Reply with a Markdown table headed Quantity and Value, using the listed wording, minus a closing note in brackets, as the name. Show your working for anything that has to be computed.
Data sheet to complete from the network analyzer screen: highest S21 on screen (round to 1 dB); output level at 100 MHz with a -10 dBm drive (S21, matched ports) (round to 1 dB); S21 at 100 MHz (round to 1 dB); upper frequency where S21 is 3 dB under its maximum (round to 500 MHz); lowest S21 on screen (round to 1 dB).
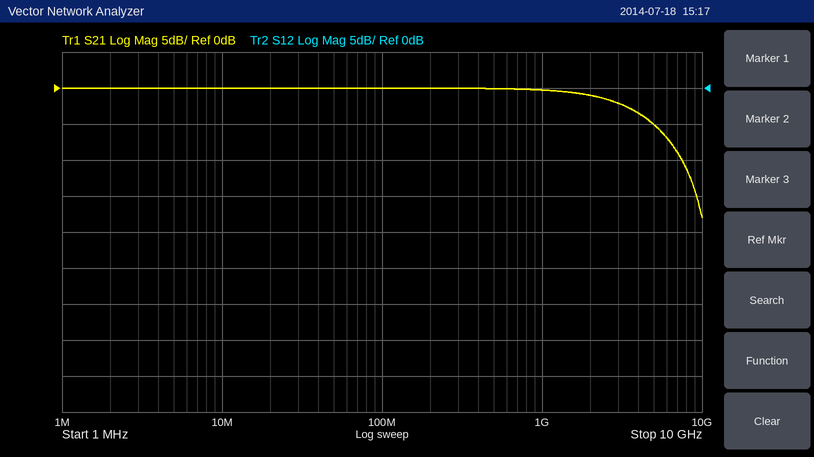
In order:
| Quantity | Value |
|---|---|
| highest S21 on screen | 0 dB |
| output level at 100 MHz with a -10 dBm drive (S21, matched ports) | -10 dBm + (0 dB) = -10 dBm |
| S21 at 100 MHz | 0 dB |
| upper frequency where S21 is 3 dB under its maximum | 3.5 GHz |
| lowest S21 on screen | -18 dB |
